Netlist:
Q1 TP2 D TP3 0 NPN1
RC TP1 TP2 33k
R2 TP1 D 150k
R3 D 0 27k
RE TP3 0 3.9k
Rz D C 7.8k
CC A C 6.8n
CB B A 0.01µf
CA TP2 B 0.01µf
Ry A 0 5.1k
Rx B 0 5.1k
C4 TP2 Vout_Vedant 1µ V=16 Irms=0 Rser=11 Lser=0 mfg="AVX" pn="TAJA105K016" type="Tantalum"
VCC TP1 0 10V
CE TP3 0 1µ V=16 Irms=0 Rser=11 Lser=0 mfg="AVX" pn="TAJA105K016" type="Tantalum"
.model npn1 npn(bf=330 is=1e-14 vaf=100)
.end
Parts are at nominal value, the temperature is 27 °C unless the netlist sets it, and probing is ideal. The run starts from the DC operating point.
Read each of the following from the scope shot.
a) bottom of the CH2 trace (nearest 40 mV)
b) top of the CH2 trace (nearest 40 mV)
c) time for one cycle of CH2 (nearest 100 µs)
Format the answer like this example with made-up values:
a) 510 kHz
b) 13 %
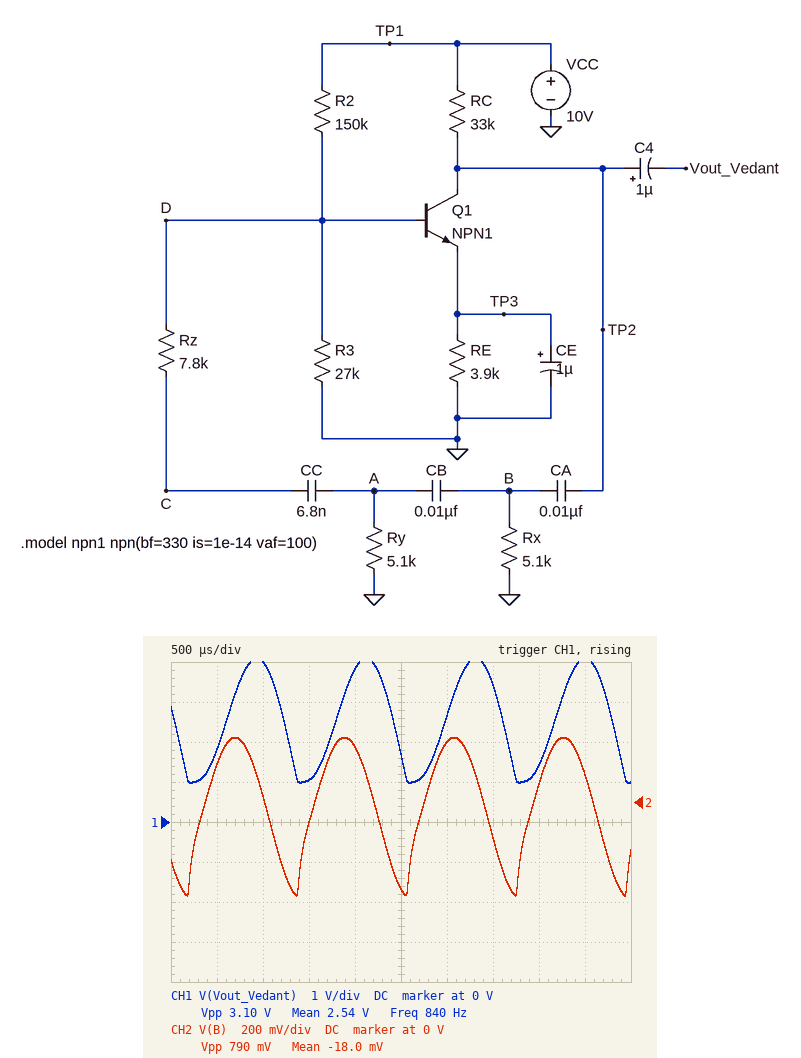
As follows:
a) -480 mV
b) 320 mV
c) 1.2 ms
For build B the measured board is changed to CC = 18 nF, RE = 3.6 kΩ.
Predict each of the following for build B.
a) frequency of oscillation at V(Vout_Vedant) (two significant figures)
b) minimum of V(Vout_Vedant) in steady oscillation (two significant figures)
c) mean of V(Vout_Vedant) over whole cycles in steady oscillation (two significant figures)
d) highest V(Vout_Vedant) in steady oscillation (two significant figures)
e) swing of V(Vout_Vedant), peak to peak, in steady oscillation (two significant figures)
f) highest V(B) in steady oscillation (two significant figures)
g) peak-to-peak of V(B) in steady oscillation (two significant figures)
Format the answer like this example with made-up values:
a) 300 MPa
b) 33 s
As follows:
a) 650 Hz
b) 1.0 V
c) 1.9 V
d) 2.8 V
e) 1.8 V
f) 150 mV
g) 350 mV
